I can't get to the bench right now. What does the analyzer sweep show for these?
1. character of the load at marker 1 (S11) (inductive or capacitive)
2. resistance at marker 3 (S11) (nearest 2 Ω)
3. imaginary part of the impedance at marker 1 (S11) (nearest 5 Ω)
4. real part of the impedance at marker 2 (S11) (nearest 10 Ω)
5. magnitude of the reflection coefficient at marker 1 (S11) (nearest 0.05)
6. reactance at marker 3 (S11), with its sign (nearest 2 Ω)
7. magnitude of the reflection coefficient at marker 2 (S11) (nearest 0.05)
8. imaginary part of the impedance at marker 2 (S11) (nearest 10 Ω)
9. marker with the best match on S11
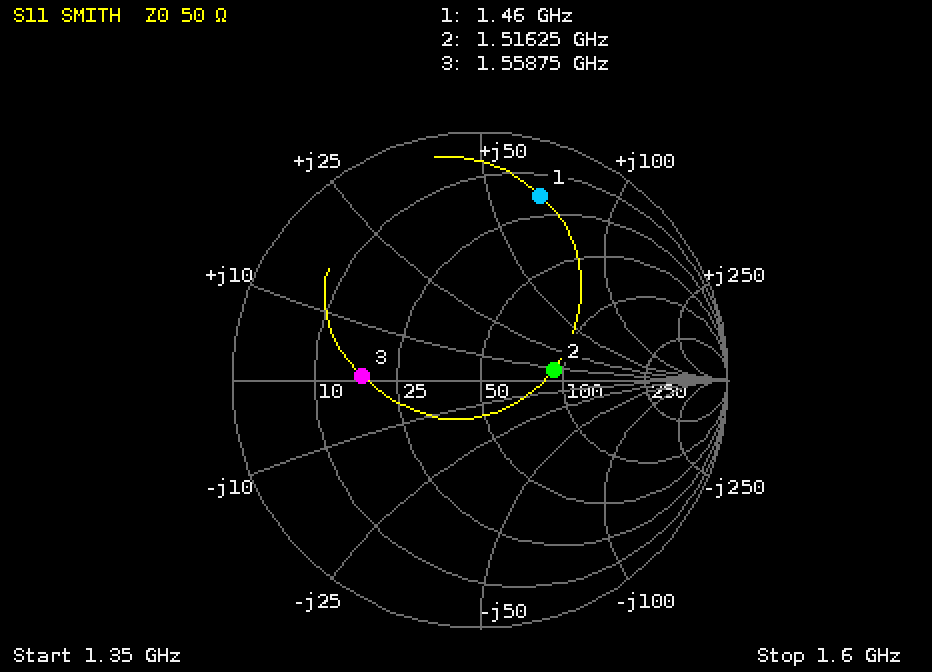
inductive
18 Ω
+65 Ω
90 Ω
0.80
0 Ω
0.30
+10 Ω
marker 2
